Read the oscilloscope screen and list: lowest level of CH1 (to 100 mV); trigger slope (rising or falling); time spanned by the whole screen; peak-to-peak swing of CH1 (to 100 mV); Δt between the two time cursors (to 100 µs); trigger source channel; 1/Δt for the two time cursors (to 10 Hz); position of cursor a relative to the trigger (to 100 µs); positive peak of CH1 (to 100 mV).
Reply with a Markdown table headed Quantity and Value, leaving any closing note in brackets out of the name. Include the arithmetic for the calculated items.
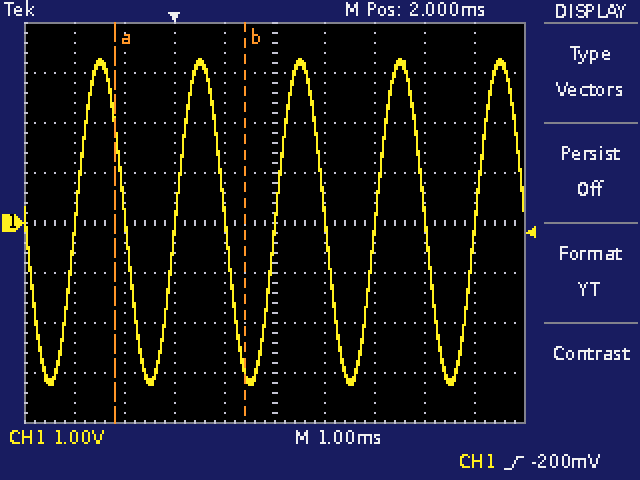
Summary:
| Quantity | Value |
|---|---|
| lowest level of CH1 | -3.2 V |
| trigger slope | rising |
| time spanned by the whole screen | 10 ms |
| peak-to-peak swing of CH1 | 3.3 V − (-3.2 V) = 6.5 V |
| Δt between the two time cursors | 2.6 ms |
| trigger source channel | CH1 |
| 1/Δt for the two time cursors | 1 / 2.6 ms ≈ 380 Hz |
| position of cursor a relative to the trigger | -1.2 ms |
| positive peak of CH1 | 3.3 V |
